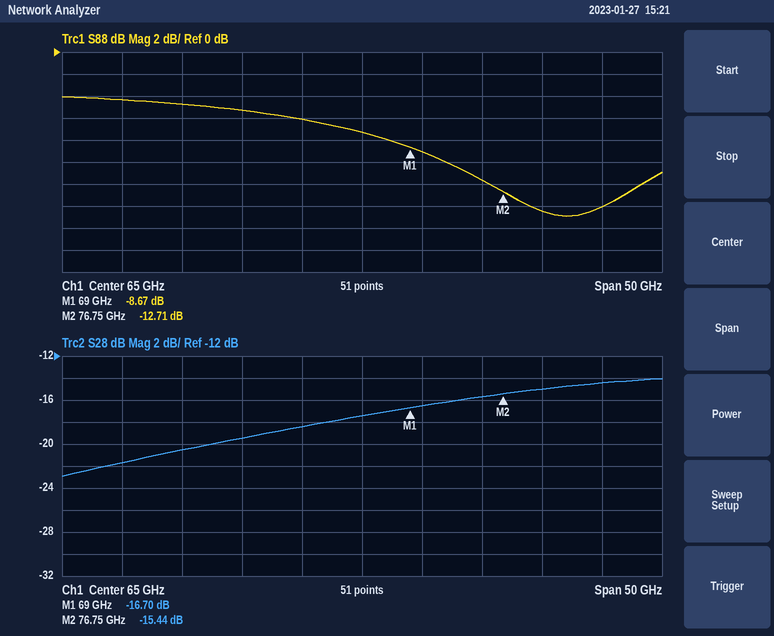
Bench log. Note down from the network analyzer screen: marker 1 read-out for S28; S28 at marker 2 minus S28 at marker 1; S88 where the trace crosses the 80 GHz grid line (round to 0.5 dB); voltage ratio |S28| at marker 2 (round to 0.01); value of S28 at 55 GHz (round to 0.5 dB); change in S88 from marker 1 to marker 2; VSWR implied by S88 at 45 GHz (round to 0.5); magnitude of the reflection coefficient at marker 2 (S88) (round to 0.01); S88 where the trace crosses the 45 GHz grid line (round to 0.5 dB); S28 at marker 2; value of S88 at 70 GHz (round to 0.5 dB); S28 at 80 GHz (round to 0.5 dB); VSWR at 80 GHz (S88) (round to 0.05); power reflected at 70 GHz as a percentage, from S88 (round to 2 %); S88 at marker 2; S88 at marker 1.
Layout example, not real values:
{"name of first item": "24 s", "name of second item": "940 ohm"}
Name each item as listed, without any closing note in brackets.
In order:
{"marker 1 read-out for S28": "-16.70 dB", "S28 at marker 2 minus S28 at marker 1": "1.26 dB", "S88 where the trace crosses the 80 GHz grid line": "-14.5 dB", "voltage ratio |S28| at marker 2": "0.17", "value of S28 at 55 GHz": "-19.5 dB", "change in S88 from marker 1 to marker 2": "-4.04 dB", "VSWR implied by S88 at 45 GHz": "4.0", "magnitude of the reflection coefficient at marker 2 (S88)": "0.23", "S88 where the trace crosses the 45 GHz grid line": "-4.5 dB", "S28 at marker 2": "-15.44 dB", "value of S88 at 70 GHz": "-9.0 dB", "S28 at 80 GHz": "-15.0 dB", "VSWR at 80 GHz (S88)": "1.45", "power reflected at 70 GHz as a percentage, from S88": "12 %", "S88 at marker 2": "-12.71 dB", "S88 at marker 1": "-8.67 dB"}
